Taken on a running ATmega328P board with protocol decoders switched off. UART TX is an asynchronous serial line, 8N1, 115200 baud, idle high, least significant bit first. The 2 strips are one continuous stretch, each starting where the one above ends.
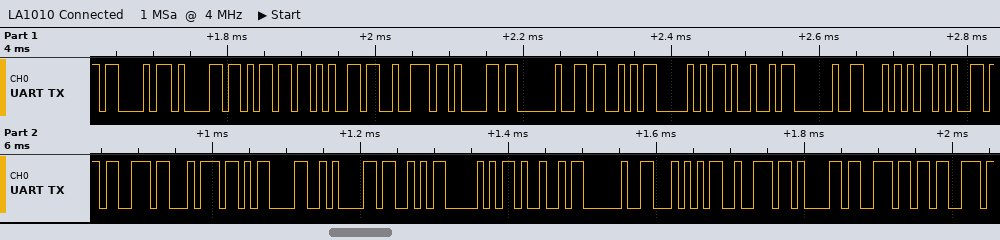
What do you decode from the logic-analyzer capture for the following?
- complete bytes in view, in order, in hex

43 61 6D 65 72 61 20 53 50 49 20 54 65 73 74 0D 0A 53 50 49 20 54 72 61 6E 73
